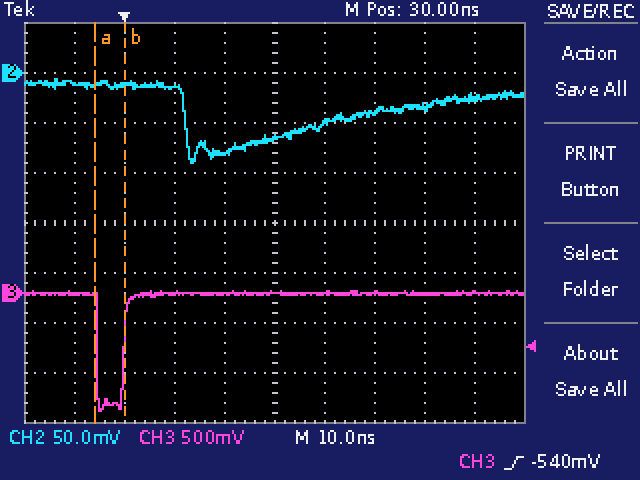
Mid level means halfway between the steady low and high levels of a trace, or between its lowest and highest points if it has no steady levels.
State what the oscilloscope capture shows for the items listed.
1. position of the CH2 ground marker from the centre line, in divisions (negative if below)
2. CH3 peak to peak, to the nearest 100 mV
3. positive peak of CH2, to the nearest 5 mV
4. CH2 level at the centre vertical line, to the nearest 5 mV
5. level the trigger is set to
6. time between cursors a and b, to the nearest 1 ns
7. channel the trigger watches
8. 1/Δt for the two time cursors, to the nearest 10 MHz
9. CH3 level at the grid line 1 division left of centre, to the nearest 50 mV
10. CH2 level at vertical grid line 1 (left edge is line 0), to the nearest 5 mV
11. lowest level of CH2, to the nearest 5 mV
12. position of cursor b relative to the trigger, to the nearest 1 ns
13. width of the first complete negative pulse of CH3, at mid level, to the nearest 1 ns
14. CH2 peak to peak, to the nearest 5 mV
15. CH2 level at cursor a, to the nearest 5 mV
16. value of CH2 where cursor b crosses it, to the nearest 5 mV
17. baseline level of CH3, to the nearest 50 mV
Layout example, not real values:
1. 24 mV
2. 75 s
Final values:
1. +3.0 div
2. 1.20 V
3. -5 mV
4. -65 mV
5. -540 mV
6. 6 ns
7. CH3
8. 170 MHz
9. 0 mV
10. -10 mV
11. -90 mV
12. 0 ns
13. 5 ns
14. 85 mV
15. -10 mV
16. -10 mV
17. 0 mV
